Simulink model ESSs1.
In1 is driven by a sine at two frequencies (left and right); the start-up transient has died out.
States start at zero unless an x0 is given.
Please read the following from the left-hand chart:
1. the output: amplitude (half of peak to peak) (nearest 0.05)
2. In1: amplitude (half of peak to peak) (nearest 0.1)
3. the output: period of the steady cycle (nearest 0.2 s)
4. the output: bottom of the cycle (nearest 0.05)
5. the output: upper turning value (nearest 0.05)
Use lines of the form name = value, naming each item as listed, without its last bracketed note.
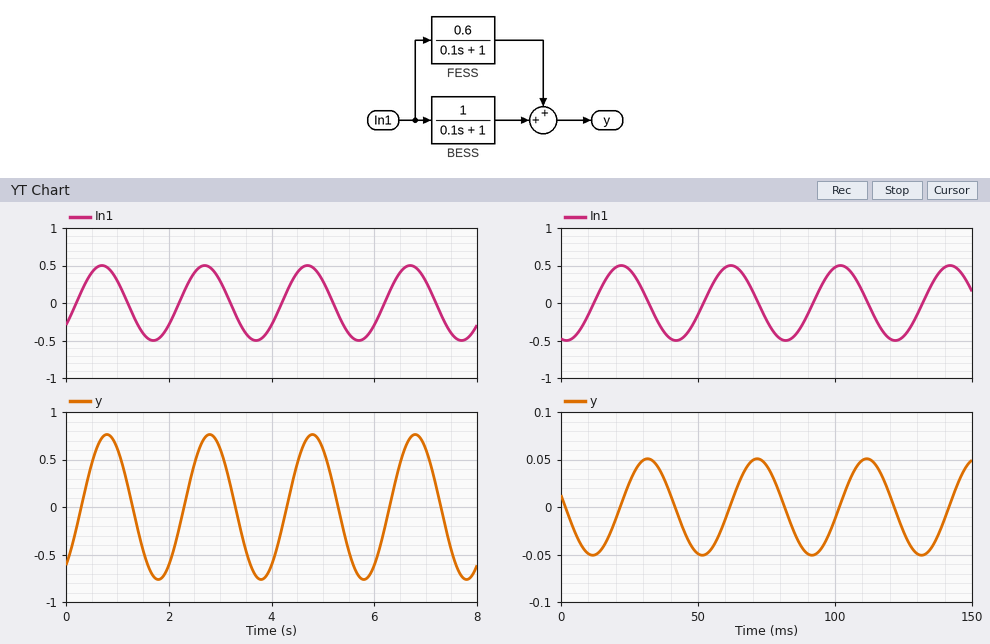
the output: amplitude (half of peak to peak) = 0.75
In1: amplitude (half of peak to peak) = 0.5
the output: period of the steady cycle = 2.0 s
the output: bottom of the cycle = -0.75
the output: upper turning value = 0.75
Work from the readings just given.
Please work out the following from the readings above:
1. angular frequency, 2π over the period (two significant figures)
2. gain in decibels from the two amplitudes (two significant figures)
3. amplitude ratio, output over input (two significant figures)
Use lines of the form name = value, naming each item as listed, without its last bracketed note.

angular frequency, 2π over the period = 3.1 rad/s
gain in decibels from the two amplitudes = 3.5 dB
amplitude ratio, output over input = 1.5
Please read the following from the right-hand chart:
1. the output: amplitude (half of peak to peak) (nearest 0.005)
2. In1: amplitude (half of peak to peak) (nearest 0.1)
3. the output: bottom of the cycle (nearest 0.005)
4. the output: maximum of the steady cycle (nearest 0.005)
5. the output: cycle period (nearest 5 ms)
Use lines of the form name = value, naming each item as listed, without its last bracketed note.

the output: amplitude (half of peak to peak) = 0.050
In1: amplitude (half of peak to peak) = 0.5
the output: bottom of the cycle = -0.050
the output: maximum of the steady cycle = 0.050
the output: cycle period = 40 ms
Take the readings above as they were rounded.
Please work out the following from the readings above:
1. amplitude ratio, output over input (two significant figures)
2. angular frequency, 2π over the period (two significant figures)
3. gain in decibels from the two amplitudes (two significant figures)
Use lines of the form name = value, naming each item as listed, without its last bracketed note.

amplitude ratio, output over input = 0.10
angular frequency, 2π over the period = 0.16 rad/ms
gain in decibels from the two amplitudes = -20 dB
